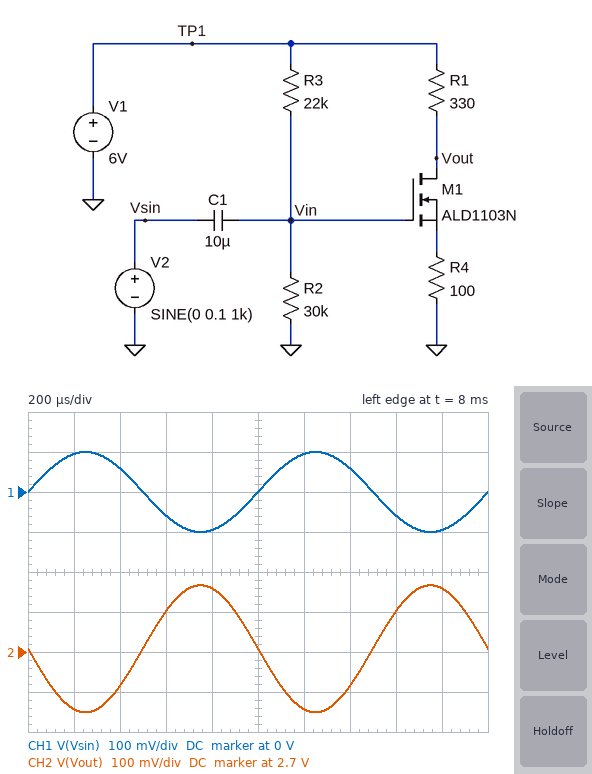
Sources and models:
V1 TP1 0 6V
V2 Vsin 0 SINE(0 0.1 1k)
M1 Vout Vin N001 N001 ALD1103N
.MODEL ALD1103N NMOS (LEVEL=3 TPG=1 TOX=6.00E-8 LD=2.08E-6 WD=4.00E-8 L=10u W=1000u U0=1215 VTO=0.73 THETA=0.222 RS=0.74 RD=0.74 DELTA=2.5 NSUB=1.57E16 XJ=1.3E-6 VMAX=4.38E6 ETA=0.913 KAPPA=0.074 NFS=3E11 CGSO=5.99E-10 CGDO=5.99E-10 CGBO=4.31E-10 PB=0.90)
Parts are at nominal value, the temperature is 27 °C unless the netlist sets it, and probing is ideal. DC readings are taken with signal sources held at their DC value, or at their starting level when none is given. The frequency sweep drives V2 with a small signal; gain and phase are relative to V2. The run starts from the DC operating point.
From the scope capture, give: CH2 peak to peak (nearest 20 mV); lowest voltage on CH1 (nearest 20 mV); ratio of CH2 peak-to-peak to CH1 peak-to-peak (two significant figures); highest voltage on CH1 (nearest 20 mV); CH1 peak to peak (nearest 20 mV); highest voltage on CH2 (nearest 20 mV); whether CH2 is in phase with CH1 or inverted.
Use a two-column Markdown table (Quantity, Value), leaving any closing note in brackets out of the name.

| Quantity | Value |
|---|---|
| CH2 peak to peak | 320 mV |
| lowest voltage on CH1 | -100 mV |
| ratio of CH2 peak-to-peak to CH1 peak-to-peak | 1.6 |
| highest voltage on CH1 | 100 mV |
| CH1 peak to peak | 200 mV |
| highest voltage on CH2 | 2.86 V |
| whether CH2 is in phase with CH1 or inverted | inverted |
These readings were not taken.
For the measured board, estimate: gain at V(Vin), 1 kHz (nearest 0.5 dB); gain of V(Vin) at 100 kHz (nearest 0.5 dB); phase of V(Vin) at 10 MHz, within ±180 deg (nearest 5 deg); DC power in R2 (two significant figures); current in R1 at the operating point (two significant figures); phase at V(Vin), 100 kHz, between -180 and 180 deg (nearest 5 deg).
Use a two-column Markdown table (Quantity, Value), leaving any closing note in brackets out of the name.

| Quantity | Value |
|---|---|
| gain at V(Vin), 1 kHz | 0 dB |
| gain of V(Vin) at 100 kHz | 0 dB |
| phase of V(Vin) at 10 MHz, within ±180 deg | 0 deg |
| DC power in R2 | 400 µW |
| current in R1 at the operating point | 10 mA |
| phase at V(Vin), 100 kHz, between -180 and 180 deg | 0 deg |
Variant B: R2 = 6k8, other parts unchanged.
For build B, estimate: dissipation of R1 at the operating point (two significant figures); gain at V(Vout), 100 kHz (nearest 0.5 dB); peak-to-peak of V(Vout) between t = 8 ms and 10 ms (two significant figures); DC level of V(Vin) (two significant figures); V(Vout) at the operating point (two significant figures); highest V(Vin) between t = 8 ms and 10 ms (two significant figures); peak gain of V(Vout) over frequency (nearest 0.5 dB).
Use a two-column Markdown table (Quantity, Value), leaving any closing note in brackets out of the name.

| Quantity | Value |
|---|---|
| dissipation of R1 at the operating point | 720 µW |
| gain at V(Vout), 100 kHz | 0 dB |
| peak-to-peak of V(Vout) between t = 8 ms and 10 ms | 200 mV |
| DC level of V(Vin) | 1.4 V |
| V(Vout) at the operating point | 5.5 V |
| highest V(Vin) between t = 8 ms and 10 ms | 1.5 V |
| peak gain of V(Vout) over frequency | 1.0 dB |
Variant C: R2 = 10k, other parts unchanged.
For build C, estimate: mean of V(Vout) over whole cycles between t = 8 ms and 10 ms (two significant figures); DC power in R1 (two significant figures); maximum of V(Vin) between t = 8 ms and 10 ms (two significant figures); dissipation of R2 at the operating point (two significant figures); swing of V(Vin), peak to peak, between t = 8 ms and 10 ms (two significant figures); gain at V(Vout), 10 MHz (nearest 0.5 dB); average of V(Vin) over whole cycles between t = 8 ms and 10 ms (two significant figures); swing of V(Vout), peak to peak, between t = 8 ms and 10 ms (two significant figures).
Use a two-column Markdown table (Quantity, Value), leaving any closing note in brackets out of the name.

| Quantity | Value |
|---|---|
| mean of V(Vout) over whole cycles between t = 8 ms and 10 ms | 5.0 V |
| DC power in R1 | 3.1 mW |
| maximum of V(Vin) between t = 8 ms and 10 ms | 2.0 V |
| dissipation of R2 at the operating point | 350 µW |
| swing of V(Vin), peak to peak, between t = 8 ms and 10 ms | 200 mV |
| gain at V(Vout), 10 MHz | 2.0 dB |
| average of V(Vin) over whole cycles between t = 8 ms and 10 ms | 1.9 V |
| swing of V(Vout), peak to peak, between t = 8 ms and 10 ms | 250 mV |
